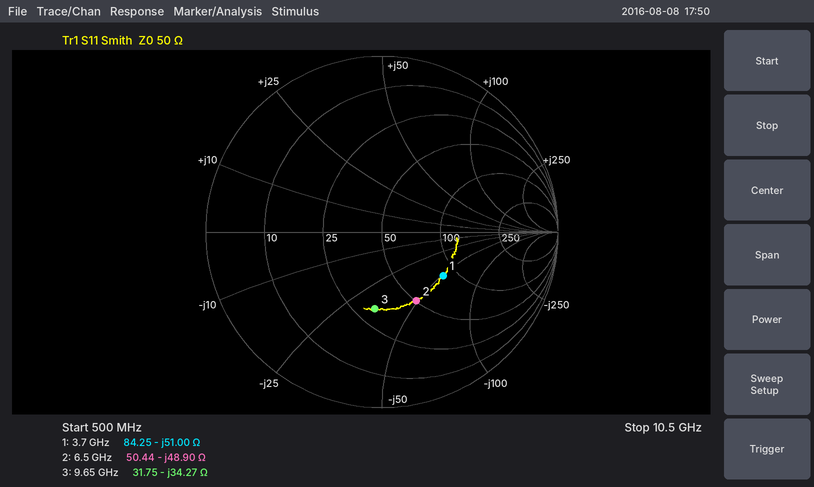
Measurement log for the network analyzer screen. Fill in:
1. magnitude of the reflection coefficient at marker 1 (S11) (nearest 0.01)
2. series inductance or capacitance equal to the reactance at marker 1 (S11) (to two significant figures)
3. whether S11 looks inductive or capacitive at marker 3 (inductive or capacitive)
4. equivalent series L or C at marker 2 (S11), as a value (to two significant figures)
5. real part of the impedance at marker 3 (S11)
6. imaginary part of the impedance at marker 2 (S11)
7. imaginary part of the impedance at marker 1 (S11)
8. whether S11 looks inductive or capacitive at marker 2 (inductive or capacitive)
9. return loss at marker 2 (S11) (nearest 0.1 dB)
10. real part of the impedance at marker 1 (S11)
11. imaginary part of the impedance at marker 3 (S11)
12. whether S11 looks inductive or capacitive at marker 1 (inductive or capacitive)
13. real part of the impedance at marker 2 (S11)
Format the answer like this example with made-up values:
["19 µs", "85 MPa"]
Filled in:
["0.43", "840 fF", "capacitive", "500 fF", "31.75 Ω", "-48.90 Ω", "-51.00 Ω", "capacitive", "7.2 dB", "84.25 Ω", "-34.27 Ω", "capacitive", "50.44 Ω"]
